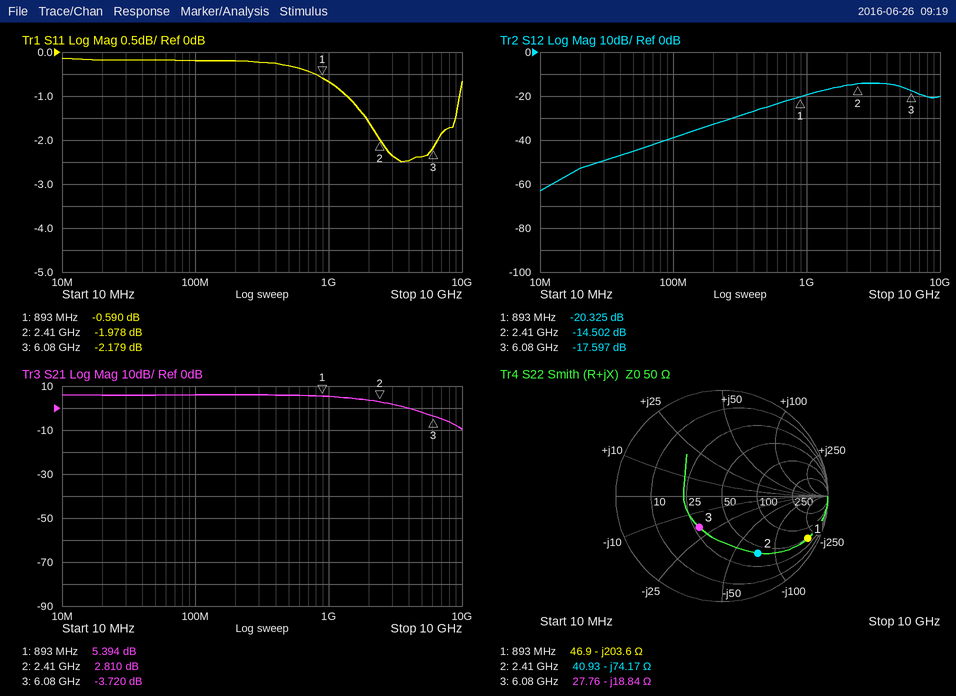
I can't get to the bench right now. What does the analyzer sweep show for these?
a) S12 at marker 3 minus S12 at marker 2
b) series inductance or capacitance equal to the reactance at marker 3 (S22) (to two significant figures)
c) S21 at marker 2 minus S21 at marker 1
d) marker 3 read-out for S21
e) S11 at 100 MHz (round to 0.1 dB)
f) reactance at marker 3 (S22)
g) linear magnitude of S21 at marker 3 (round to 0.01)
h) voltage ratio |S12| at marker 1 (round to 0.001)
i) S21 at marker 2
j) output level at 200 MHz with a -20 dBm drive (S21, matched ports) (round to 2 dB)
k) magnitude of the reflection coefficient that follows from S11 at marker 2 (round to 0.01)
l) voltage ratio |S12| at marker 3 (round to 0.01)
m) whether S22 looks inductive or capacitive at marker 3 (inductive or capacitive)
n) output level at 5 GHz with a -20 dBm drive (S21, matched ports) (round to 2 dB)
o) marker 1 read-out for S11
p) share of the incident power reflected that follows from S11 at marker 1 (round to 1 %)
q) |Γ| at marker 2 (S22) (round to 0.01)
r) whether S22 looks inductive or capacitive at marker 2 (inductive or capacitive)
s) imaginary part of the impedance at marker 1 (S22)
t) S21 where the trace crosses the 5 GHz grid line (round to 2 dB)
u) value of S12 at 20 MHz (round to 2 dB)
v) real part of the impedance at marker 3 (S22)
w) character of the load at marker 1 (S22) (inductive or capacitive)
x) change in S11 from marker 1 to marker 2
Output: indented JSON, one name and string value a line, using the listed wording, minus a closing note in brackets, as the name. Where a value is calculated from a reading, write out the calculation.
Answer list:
{
  "S12 at marker 3 minus S12 at marker 2": "-17.597 − (-14.502) = -3.095 dB",
  "series inductance or capacitance equal to the reactance at marker 3 (S22)": "C = 1/(2π × 6.08 GHz × 18.84 Ω) ≈ 1.4 pF",
  "S21 at marker 2 minus S21 at marker 1": "2.81 − (5.394) = -2.584 dB",
  "marker 3 read-out for S21": "-3.720 dB",
  "S11 at 100 MHz": "-0.2 dB",
  "reactance at marker 3": "-18.84 Ω",
  "linear magnitude of S21 at marker 3": "10^(-3.72/20) ≈ 0.65",
  "voltage ratio |S12| at marker 1": "10^(-20.325/20) ≈ 0.096",
  "S21 at marker 2": "2.810 dB",
  "output level at 200 MHz with a -20 dBm drive (S21, matched ports)": "-20 dBm + (6 dB) = -14 dBm",
  "magnitude of the reflection coefficient that follows from S11 at marker 2": "10^(-1.978/20) ≈ 0.80",
  "voltage ratio |S12| at marker 3": "10^(-17.597/20) ≈ 0.13",
  "whether S22 looks inductive or capacitive at marker 3": "capacitive",
  "output level at 5 GHz with a -20 dBm drive (S21, matched ports)": "-20 dBm + (-2 dB) = -22 dBm",
  "marker 1 read-out for S11": "-0.590 dB",
  "share of the incident power reflected that follows from S11 at marker 1": "10^(-0.59/10) ≈ 87 %",
  "|Γ| at marker 2 (S22)": "0.64",
  "whether S22 looks inductive or capacitive at marker 2": "capacitive",
  "imaginary part of the impedance at marker 1": "-203.6 Ω",
  "S21 where the trace crosses the 5 GHz grid line": "-2 dB",
  "value of S12 at 20 MHz": "-52 dB",
  "real part of the impedance at marker 3": "27.76 Ω",
  "character of the load at marker 1 (S22)": "capacitive",
  "change in S11 from marker 1 to marker 2": "-1.978 − (-0.59) = -1.388 dB"
}
